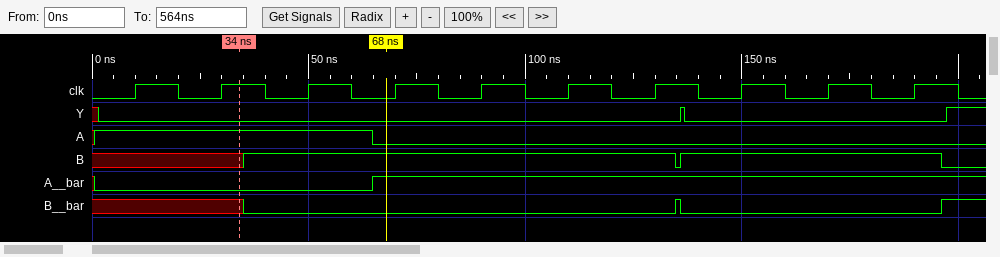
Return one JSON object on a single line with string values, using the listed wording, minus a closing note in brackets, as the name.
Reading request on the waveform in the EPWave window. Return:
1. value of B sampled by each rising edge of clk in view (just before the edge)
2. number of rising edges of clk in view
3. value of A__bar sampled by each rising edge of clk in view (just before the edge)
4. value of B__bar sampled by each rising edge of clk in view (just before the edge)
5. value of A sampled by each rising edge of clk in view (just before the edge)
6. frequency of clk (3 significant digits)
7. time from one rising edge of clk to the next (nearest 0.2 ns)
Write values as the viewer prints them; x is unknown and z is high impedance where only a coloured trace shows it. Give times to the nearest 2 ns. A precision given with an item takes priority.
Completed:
{"value of B sampled by each rising edge of clk in view": "x x 1 1 1 1 1 1 1 1", "number of rising edges of clk in view": "10", "value of A__bar sampled by each rising edge of clk in view": "0 0 0 1 1 1 1 1 1 1", "value of B__bar sampled by each rising edge of clk in view": "x x 0 0 0 0 0 0 0 0", "value of A sampled by each rising edge of clk in view": "1 1 1 0 0 0 0 0 0 0", "frequency of clk": "50.0 MHz", "time from one rising edge of clk to the next": "20 ns"}
